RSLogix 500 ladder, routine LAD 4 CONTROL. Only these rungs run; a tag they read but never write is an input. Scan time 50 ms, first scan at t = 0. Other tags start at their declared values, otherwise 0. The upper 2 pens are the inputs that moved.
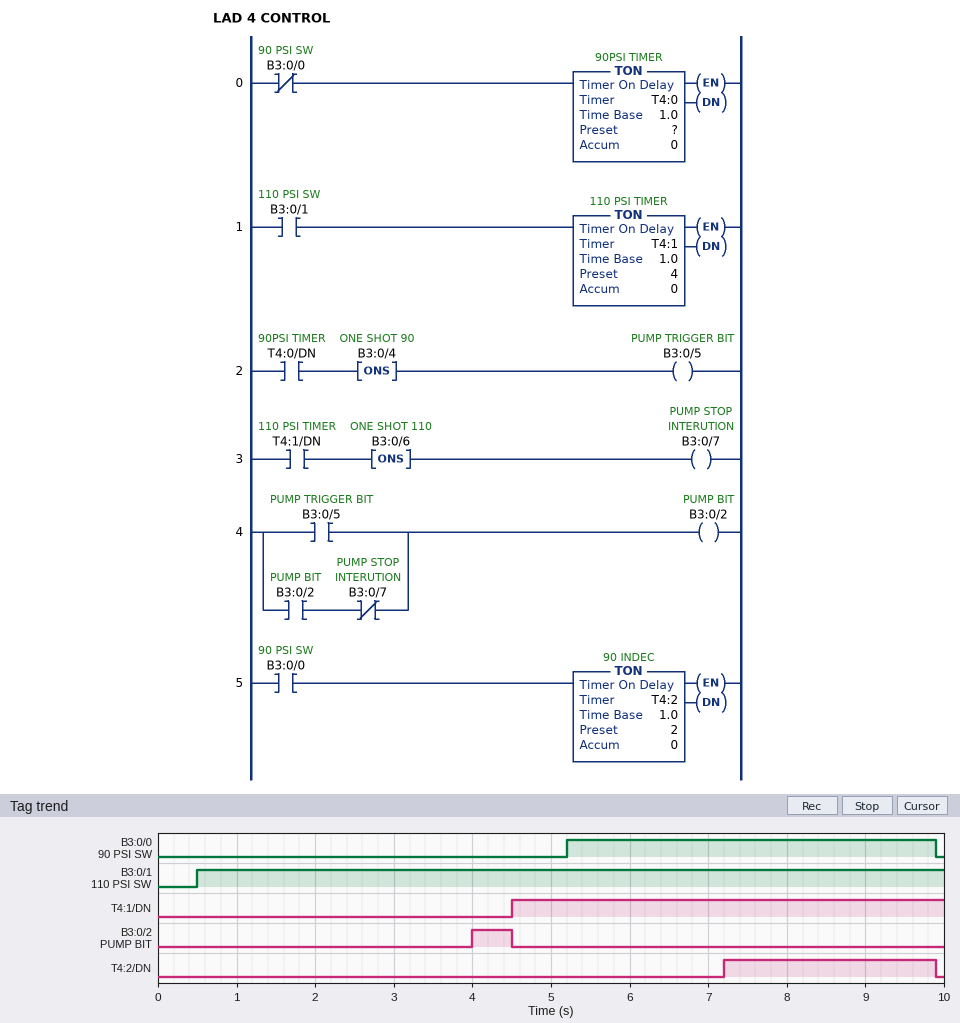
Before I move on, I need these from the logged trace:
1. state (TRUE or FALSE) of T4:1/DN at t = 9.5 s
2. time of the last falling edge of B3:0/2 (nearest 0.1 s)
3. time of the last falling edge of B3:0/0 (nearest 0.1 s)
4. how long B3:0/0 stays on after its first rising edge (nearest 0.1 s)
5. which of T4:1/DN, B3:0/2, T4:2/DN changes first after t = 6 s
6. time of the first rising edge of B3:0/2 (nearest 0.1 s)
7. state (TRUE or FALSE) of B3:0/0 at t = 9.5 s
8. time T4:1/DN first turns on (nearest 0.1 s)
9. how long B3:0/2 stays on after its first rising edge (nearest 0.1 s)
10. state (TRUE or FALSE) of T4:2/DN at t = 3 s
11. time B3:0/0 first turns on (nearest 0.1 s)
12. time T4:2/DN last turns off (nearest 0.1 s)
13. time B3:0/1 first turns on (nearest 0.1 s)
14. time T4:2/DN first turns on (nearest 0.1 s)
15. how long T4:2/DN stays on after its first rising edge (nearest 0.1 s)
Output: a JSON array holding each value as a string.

["TRUE", "4.5 s", "9.9 s", "4.7 s", "T4:2/DN", "4.0 s", "TRUE", "4.5 s", "0.5 s", "FALSE", "5.2 s", "9.9 s", "0.5 s", "7.2 s", "2.7 s"]
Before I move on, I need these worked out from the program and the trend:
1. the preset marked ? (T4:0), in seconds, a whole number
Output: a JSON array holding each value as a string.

["4 s"]
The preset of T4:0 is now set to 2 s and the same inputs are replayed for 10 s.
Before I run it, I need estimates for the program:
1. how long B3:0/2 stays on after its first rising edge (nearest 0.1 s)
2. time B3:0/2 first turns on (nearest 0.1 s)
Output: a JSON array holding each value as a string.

["2.5 s", "2.0 s"]
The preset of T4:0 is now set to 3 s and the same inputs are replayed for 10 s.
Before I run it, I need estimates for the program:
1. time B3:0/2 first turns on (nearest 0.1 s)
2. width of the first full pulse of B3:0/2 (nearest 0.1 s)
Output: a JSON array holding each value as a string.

["3.0 s", "1.5 s"]
